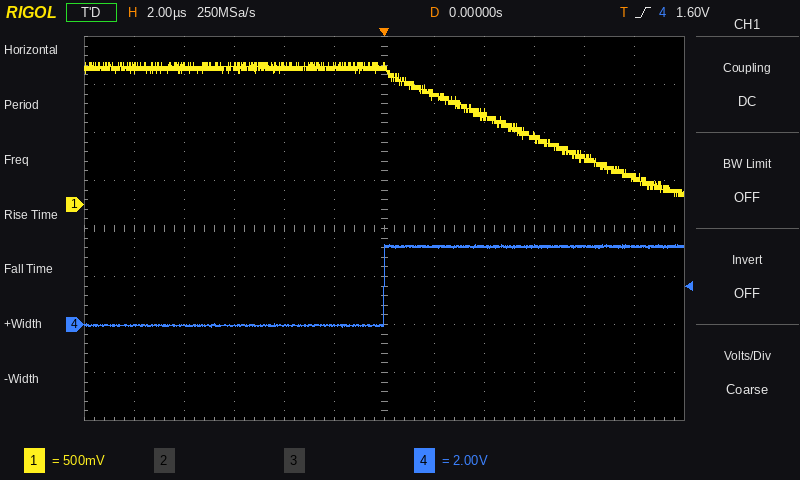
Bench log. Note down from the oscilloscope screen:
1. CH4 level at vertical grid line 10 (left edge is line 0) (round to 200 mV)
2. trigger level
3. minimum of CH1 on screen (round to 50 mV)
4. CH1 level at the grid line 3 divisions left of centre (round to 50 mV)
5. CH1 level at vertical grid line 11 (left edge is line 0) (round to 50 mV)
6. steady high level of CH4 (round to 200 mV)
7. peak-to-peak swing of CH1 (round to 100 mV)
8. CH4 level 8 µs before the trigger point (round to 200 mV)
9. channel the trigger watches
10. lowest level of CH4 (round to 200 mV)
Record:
3.2 V
1.60 V
100 mV
1.45 V
300 mV
3.2 V
1.40 V
0.0 V
CH4
-200 mV
